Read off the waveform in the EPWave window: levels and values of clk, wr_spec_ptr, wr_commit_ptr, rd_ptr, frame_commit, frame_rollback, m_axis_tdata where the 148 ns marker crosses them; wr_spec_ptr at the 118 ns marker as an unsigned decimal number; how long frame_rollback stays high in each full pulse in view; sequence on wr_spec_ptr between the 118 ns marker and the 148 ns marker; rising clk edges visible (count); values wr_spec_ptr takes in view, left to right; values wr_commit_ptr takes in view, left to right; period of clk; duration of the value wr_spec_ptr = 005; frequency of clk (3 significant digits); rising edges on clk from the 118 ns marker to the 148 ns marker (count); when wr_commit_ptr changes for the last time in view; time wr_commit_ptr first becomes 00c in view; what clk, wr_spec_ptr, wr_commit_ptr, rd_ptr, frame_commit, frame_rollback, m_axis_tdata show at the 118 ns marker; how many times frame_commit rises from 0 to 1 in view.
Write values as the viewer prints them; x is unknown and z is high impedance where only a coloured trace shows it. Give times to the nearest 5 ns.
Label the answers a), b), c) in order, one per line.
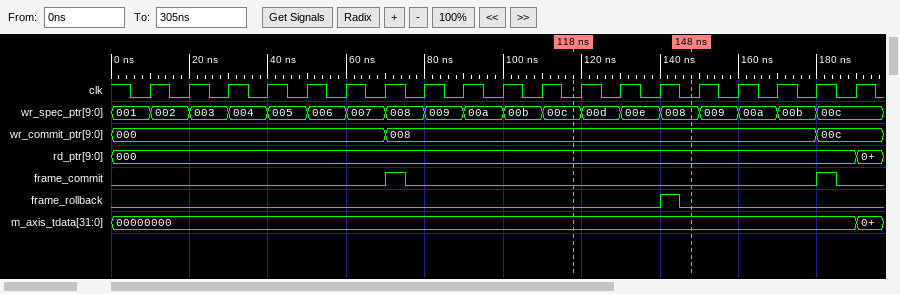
a) clk=0, wr_spec_ptr=008, wr_commit_ptr=008, rd_ptr=000, frame_commit=0, frame_rollback=0, m_axis_tdata=00000000
b) 12
c) 5 ns
d) 00c, 00d, 00e, 008
e) 19
f) 001, 002, 003, 004, 005, 006, 007, 008, 009, 00a, 00b, 00c, 00d, 00e, 008, 009, 00a, 00b, 00c
g) 000, 008, 00c
h) 10 ns
i) 10 ns
j) 100 MHz
k) 3
l) 180 ns
m) 180 ns
n) clk=0, wr_spec_ptr=00c, wr_commit_ptr=008, rd_ptr=000, frame_commit=0, frame_rollback=0, m_axis_tdata=00000000
o) 2
